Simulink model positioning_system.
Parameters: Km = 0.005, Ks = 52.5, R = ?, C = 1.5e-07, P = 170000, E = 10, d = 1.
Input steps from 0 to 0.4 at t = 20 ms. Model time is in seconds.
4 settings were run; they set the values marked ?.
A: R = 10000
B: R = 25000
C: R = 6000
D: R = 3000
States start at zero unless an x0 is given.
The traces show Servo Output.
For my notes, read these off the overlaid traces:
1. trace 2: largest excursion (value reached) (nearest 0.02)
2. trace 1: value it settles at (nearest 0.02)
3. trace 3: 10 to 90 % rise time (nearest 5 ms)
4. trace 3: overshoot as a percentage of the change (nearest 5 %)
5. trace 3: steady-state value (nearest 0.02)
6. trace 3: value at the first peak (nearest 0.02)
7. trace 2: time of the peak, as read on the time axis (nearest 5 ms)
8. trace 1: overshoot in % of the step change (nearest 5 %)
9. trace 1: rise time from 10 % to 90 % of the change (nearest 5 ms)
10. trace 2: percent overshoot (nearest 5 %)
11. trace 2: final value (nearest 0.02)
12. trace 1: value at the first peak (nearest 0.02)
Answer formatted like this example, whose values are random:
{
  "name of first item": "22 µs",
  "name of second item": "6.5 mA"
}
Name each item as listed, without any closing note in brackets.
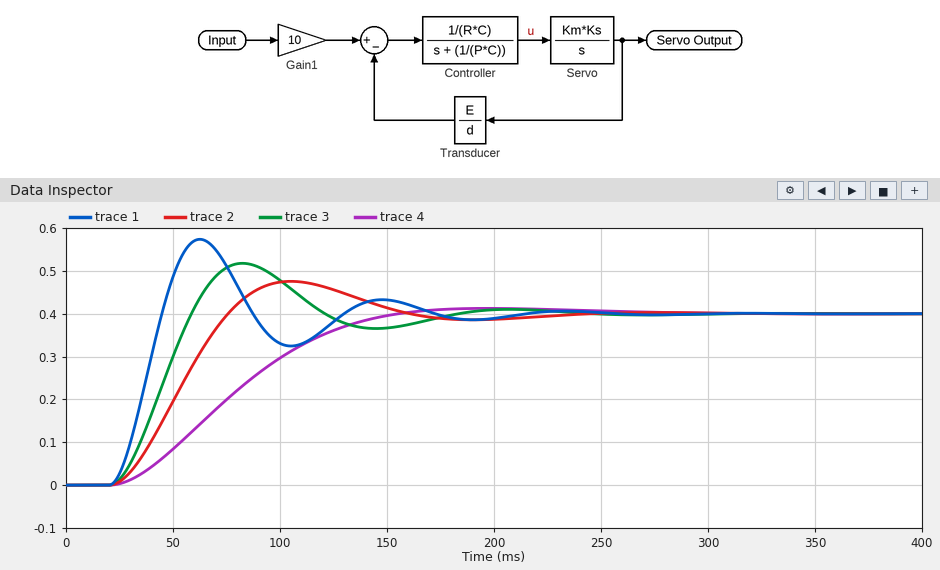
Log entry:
{
  "trace 2: largest excursion (value reached)": "0.48",
  "trace 1: value it settles at": "0.40",
  "trace 3: 10 to 90 % rise time": "25 ms",
  "trace 3: overshoot as a percentage of the change": "30 %",
  "trace 3: steady-state value": "0.40",
  "trace 3: value at the first peak": "0.52",
  "trace 2: time of the peak, as read on the time axis": "105 ms",
  "trace 1: overshoot in % of the step change": "45 %",
  "trace 1: rise time from 10 % to 90 % of the change": "15 ms",
  "trace 2: percent overshoot": "20 %",
  "trace 2: final value": "0.40",
  "trace 1: value at the first peak": "0.58"
}
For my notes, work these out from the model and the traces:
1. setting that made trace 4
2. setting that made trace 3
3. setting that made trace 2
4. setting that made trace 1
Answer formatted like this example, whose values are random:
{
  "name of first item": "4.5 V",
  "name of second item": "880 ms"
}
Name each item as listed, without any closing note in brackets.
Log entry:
{
  "setting that made trace 4": "B",
  "setting that made trace 3": "C",
  "setting that made trace 2": "A",
  "setting that made trace 1": "D"
}
